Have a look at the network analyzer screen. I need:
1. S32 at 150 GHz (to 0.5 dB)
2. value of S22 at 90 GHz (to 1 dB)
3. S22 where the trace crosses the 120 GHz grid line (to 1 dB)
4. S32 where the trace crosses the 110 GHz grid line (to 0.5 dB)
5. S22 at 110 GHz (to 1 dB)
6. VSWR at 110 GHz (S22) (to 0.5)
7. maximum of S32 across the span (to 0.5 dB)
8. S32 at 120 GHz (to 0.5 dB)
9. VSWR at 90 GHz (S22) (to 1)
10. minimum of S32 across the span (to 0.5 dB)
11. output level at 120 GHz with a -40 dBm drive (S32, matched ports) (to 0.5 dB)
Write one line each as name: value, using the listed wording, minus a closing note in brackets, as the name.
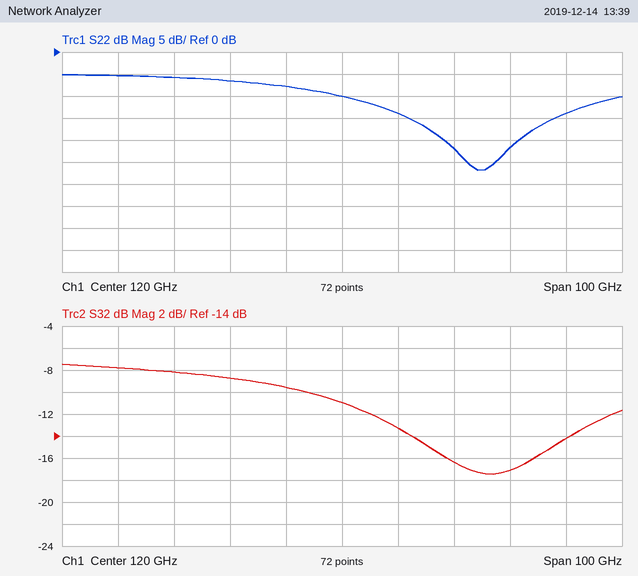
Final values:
S32 at 150 GHz: -17.0 dB
value of S22 at 90 GHz: -6 dB
S22 where the trace crosses the 120 GHz grid line: -10 dB
S32 where the trace crosses the 110 GHz grid line: -9.5 dB
S22 at 110 GHz: -8 dB
VSWR at 110 GHz (S22): 2.5
maximum of S32 across the span: -7.5 dB
S32 at 120 GHz: -11.0 dB
VSWR at 90 GHz (S22): 3
minimum of S32 across the span: -17.5 dB
output level at 120 GHz with a -40 dBm drive (S32, matched ports): -51.0 dBm
